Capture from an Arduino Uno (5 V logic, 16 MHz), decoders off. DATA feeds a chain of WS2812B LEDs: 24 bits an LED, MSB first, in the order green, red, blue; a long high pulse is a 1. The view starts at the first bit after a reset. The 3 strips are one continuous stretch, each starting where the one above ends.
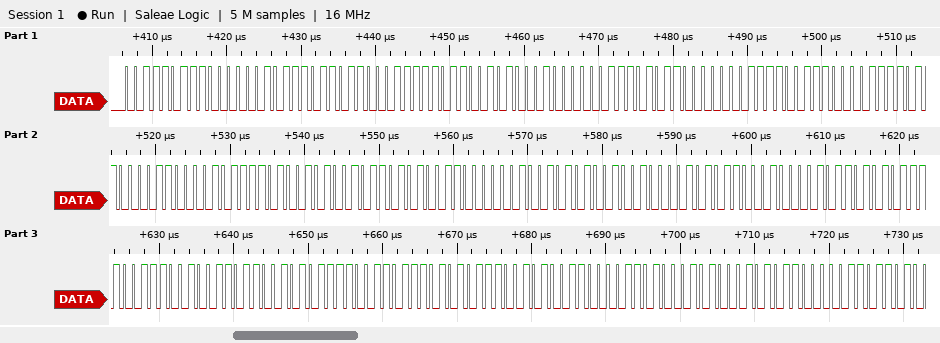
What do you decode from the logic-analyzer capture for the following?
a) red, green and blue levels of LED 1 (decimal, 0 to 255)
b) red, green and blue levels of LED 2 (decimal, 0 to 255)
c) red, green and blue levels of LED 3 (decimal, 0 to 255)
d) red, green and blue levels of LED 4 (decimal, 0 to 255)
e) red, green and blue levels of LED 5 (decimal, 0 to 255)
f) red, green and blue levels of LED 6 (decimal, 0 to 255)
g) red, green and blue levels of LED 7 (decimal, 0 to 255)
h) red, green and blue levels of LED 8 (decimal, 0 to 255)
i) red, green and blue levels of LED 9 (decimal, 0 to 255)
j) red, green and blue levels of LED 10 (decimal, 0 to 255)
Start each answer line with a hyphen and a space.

- 129, 59, 118
- 217, 199, 68
- 176, 14, 30
- 246, 112, 24
- 148, 94, 181
- 37, 48, 73
- 196, 10, 45
- 114, 94, 108
- 55, 175, 87
- 134, 41, 138
